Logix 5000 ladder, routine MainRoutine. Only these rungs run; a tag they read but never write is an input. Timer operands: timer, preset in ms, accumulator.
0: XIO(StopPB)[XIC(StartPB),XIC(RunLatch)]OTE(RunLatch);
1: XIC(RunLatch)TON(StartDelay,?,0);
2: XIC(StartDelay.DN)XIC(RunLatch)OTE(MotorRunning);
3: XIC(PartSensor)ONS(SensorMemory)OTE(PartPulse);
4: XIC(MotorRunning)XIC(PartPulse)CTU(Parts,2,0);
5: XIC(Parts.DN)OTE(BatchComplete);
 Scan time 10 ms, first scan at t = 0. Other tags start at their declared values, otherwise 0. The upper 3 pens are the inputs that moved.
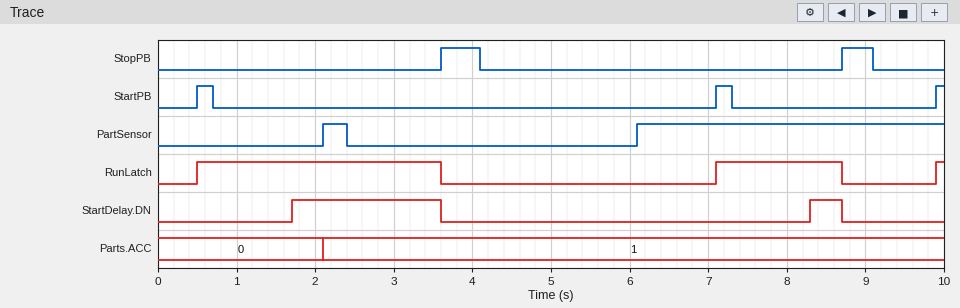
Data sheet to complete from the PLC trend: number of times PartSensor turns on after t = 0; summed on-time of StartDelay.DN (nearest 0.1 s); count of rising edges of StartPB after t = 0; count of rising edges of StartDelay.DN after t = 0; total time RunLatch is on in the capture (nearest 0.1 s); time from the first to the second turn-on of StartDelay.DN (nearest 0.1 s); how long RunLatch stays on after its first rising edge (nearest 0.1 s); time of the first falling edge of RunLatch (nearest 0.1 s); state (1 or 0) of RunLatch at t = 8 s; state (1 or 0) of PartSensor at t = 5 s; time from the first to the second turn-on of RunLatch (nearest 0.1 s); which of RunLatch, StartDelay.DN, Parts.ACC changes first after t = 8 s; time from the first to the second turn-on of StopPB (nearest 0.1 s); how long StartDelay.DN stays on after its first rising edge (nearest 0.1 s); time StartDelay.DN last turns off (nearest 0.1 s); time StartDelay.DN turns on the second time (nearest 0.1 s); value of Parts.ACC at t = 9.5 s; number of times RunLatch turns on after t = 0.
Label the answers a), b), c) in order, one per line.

a) 2
b) 2.3 s
c) 3
d) 2
e) 4.8 s
f) 6.6 s
g) 3.1 s
h) 3.6 s
i) 1
j) 0
k) 6.6 s
l) StartDelay.DN
m) 5.1 s
n) 1.9 s
o) 8.7 s
p) 8.3 s
q) 1
r) 3
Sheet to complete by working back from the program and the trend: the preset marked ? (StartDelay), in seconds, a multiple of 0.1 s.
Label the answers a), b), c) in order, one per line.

a) 1.2 s
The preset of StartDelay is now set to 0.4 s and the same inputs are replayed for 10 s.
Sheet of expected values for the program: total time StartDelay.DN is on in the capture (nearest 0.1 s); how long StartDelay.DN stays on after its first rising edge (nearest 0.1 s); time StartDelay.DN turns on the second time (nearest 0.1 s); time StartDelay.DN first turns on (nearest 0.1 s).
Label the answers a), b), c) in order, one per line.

a) 3.9 s
b) 2.7 s
c) 7.5 s
d) 0.9 s
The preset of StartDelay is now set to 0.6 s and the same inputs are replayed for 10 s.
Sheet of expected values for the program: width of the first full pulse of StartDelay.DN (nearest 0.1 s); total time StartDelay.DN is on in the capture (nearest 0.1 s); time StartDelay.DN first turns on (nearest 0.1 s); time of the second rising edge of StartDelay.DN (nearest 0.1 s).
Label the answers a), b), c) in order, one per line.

a) 2.5 s
b) 3.5 s
c) 1.1 s
d) 7.7 s
